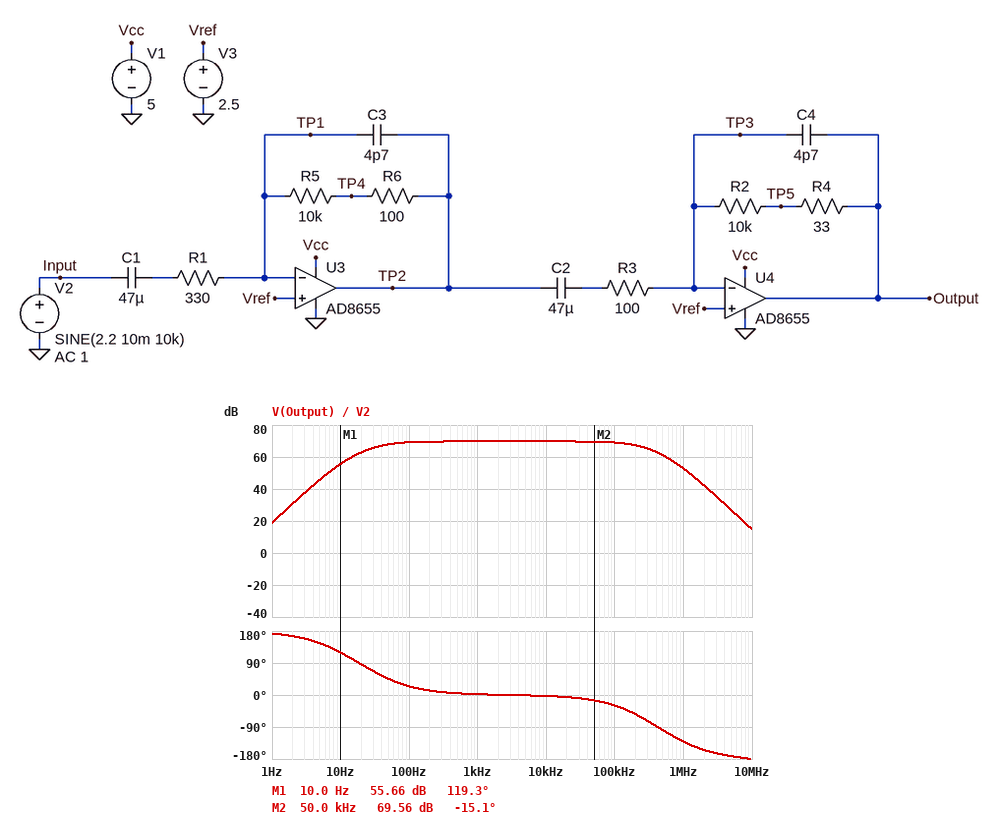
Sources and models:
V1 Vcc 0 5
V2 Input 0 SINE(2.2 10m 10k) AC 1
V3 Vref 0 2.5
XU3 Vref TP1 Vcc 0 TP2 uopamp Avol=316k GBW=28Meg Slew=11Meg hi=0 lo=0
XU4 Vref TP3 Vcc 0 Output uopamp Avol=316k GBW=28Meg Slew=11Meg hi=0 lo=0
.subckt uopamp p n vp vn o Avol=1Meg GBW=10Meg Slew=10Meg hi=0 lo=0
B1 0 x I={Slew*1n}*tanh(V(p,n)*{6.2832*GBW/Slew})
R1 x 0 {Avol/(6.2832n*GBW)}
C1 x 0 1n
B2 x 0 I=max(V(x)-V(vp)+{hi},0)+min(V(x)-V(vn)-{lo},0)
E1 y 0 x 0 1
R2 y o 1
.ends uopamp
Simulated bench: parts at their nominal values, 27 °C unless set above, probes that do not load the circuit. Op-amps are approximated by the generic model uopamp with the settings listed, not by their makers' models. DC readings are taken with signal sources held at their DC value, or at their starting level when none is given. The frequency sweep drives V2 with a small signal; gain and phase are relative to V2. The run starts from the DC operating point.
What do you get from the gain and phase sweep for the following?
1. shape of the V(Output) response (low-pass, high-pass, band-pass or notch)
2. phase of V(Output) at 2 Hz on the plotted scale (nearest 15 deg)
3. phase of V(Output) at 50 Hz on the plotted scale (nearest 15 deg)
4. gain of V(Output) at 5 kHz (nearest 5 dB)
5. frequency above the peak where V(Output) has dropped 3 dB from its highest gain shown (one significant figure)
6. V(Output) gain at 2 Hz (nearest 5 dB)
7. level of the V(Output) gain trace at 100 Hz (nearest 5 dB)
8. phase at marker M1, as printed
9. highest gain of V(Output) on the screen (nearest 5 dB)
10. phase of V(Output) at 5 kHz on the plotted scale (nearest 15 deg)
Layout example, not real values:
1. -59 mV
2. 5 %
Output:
1. band-pass
2. 165 deg
3. 45 deg
4. 70 dB
5. 200 kHz
6. 30 dB
7. 70 dB
8. 119.3 deg
9. 70 dB
10. 0 deg
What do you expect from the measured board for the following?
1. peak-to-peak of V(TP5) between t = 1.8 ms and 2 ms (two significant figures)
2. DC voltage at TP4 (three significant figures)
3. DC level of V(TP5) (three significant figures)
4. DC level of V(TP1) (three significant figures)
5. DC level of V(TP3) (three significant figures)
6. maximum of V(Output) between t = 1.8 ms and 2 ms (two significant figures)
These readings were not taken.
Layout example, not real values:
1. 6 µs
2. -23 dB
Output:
1. 5.0 V
2. 2.50 V
3. 2.50 V
4. 2.50 V
5. 2.50 V
6. 5.0 V
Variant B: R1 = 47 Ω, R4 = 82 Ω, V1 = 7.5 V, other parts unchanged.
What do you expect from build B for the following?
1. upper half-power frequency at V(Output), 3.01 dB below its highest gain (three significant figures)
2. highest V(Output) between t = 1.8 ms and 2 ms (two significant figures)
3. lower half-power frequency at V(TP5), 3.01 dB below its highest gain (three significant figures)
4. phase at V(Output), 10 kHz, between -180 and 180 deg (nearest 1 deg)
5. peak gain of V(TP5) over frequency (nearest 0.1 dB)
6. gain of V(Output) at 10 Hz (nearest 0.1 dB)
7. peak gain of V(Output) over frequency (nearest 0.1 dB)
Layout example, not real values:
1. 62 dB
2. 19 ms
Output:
1. 104 kHz
2. 7.5 V
3. 84.5 Hz
4. -6 deg
5. 86.6 dB
6. 58.5 dB
7. 86.7 dB
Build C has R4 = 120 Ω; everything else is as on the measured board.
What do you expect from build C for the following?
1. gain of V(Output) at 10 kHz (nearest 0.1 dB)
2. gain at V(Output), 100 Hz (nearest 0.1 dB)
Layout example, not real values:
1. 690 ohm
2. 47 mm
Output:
1. 69.8 dB
2. 69.3 dB
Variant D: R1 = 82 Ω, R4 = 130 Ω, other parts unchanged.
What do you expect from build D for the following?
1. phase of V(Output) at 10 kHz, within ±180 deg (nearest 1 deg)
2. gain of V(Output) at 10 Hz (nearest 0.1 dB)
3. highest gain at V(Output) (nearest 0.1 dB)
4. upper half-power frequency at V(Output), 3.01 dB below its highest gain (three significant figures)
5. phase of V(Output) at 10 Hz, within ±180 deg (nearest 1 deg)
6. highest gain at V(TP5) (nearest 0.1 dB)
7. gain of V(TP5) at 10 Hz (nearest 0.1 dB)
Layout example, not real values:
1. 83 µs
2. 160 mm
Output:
1. -5 deg
2. 58.4 dB
3. 81.9 dB
4. 147 kHz
5. 150 deg
6. 81.8 dB
7. 58.3 dB
